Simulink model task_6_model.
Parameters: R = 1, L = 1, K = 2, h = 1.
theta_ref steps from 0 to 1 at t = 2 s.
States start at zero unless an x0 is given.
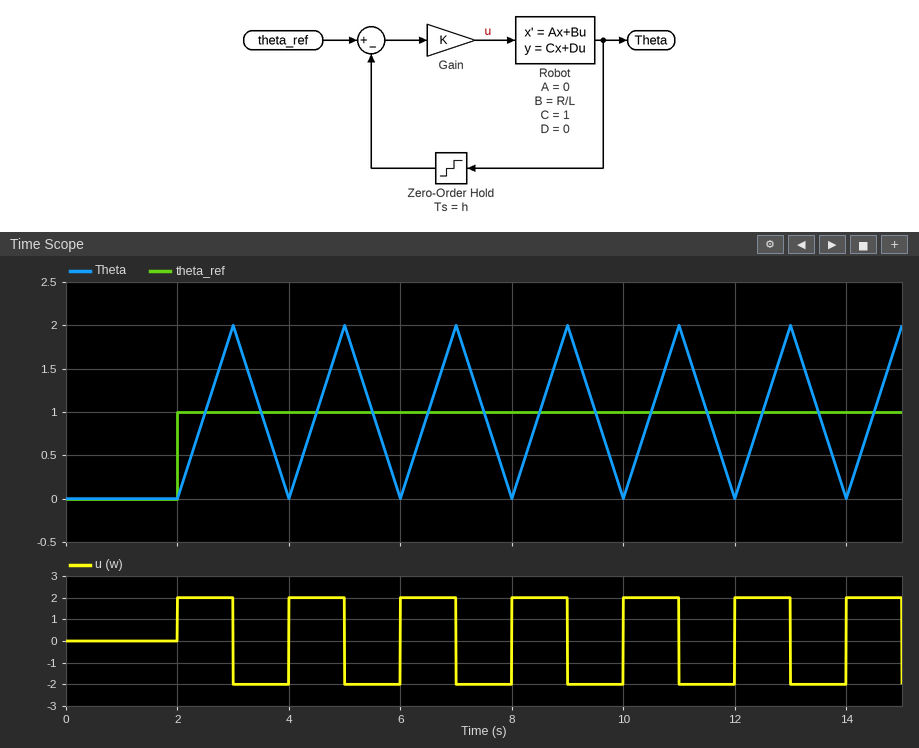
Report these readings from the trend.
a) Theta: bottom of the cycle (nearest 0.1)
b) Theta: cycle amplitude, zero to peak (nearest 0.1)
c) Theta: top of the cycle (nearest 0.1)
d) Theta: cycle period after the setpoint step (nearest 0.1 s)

0.0
1.0
2.0
2.0 s
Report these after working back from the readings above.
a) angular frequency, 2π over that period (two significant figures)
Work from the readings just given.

3.1 rad/s
